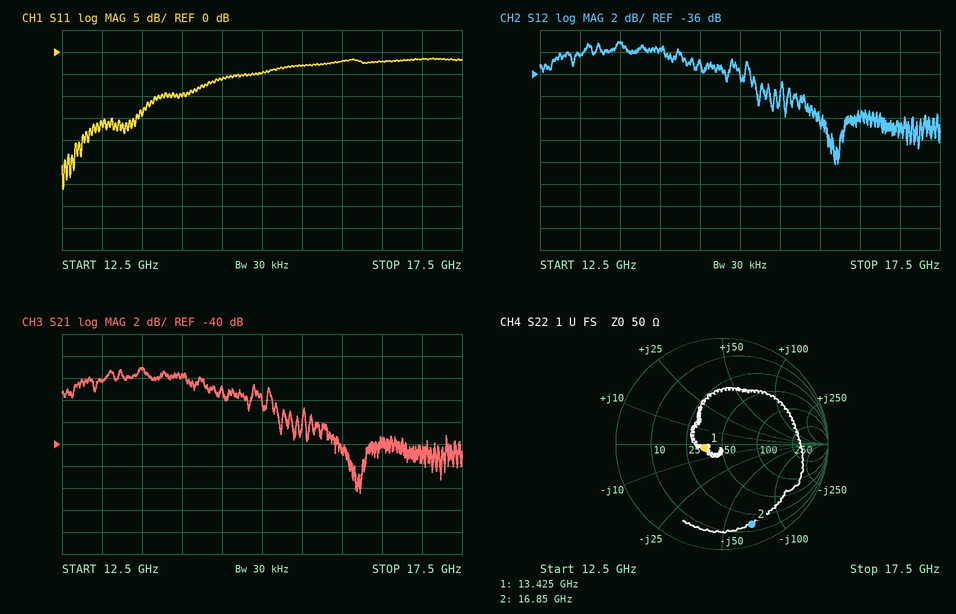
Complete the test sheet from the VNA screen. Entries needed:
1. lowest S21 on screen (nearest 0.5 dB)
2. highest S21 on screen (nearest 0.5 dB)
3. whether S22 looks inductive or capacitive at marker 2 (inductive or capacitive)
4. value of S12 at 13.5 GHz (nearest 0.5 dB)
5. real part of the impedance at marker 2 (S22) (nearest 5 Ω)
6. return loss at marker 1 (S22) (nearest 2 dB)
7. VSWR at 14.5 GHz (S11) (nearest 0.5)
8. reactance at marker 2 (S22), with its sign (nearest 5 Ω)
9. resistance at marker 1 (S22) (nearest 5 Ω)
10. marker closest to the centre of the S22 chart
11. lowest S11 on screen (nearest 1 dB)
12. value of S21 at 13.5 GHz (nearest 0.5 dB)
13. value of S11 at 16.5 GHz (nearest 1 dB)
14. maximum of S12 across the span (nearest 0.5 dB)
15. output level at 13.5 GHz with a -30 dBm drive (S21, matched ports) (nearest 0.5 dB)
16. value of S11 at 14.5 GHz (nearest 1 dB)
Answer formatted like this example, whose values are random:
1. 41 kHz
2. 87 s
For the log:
1. -44.5 dB
2. -33.0 dB
3. capacitive
4. -33.0 dB
5. 15 Ω
6. 16 dB
7. 3.0
8. -70 Ω
9. 35 Ω
10. marker 1
11. -31 dB
12. -33.0 dB
13. -2 dB
14. -33.0 dB
15. -63.0 dBm
16. -6 dB
